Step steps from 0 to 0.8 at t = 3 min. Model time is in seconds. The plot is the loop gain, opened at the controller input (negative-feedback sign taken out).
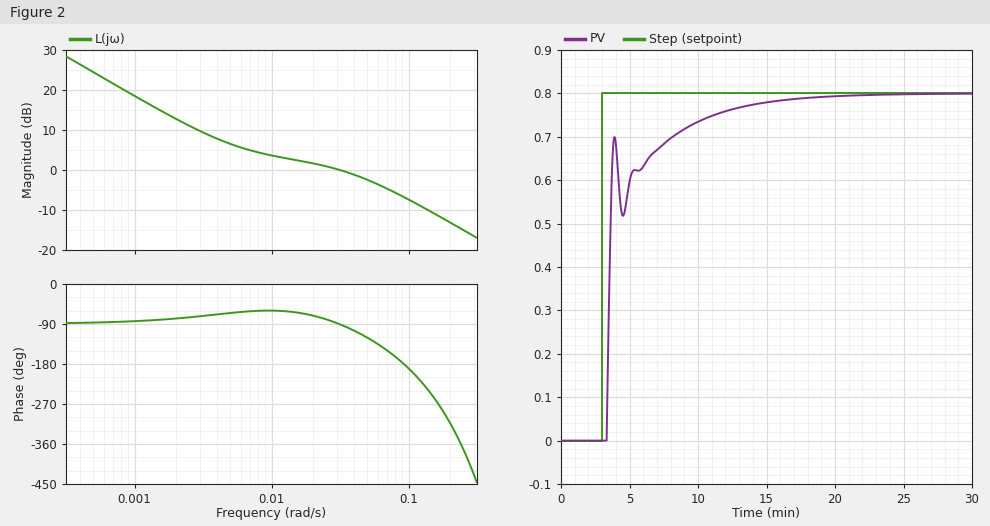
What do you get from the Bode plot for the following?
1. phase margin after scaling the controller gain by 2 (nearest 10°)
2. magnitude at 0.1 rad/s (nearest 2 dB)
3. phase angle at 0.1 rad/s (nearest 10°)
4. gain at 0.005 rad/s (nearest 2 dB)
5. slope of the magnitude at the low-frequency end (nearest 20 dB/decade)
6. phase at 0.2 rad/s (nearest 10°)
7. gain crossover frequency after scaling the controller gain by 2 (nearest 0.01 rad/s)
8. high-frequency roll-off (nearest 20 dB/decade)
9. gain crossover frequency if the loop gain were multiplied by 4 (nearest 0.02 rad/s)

10°
-8 dB
-190°
6 dB
-20 dB/decade
-310°
0.08 rad/s
-20 dB/decade
0.18 rad/s
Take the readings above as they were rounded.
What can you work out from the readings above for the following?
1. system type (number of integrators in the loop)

1
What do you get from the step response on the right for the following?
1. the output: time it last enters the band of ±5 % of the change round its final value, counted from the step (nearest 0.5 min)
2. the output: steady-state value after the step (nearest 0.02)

9.0 min
0.80
